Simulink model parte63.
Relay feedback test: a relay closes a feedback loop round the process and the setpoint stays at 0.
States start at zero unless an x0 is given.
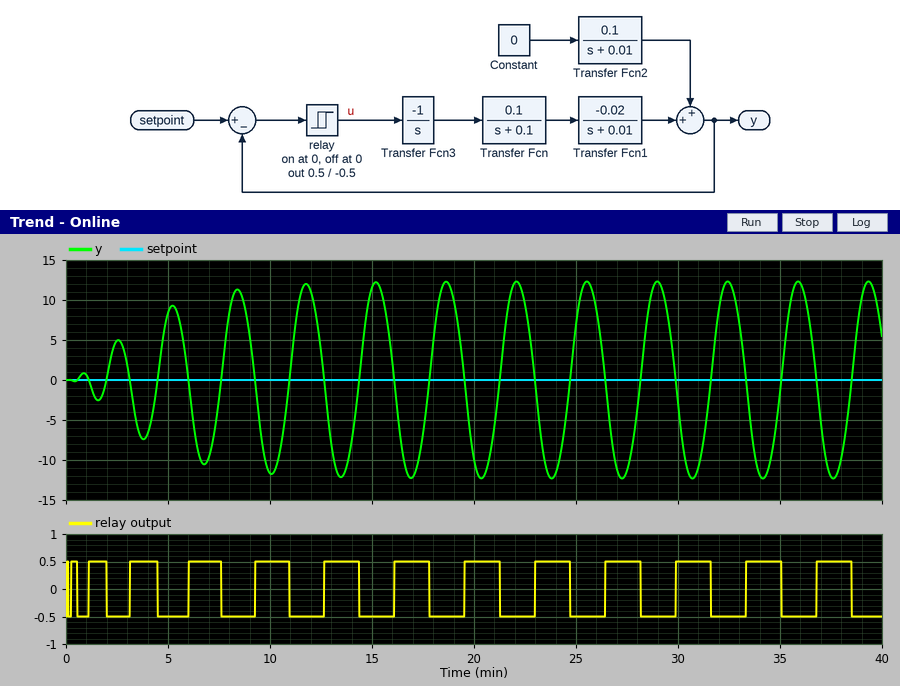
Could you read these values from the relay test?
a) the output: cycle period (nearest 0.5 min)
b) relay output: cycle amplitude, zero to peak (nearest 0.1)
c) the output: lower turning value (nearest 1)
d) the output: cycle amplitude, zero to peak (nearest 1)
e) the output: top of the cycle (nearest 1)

3.5 min
0.5
-12
12
12
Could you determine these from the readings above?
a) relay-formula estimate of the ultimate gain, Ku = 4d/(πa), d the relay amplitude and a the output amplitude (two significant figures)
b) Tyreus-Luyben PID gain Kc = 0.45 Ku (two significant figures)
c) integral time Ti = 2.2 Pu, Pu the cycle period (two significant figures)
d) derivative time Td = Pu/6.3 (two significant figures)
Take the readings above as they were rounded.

0.053
0.024
7.7 min
0.56 min
